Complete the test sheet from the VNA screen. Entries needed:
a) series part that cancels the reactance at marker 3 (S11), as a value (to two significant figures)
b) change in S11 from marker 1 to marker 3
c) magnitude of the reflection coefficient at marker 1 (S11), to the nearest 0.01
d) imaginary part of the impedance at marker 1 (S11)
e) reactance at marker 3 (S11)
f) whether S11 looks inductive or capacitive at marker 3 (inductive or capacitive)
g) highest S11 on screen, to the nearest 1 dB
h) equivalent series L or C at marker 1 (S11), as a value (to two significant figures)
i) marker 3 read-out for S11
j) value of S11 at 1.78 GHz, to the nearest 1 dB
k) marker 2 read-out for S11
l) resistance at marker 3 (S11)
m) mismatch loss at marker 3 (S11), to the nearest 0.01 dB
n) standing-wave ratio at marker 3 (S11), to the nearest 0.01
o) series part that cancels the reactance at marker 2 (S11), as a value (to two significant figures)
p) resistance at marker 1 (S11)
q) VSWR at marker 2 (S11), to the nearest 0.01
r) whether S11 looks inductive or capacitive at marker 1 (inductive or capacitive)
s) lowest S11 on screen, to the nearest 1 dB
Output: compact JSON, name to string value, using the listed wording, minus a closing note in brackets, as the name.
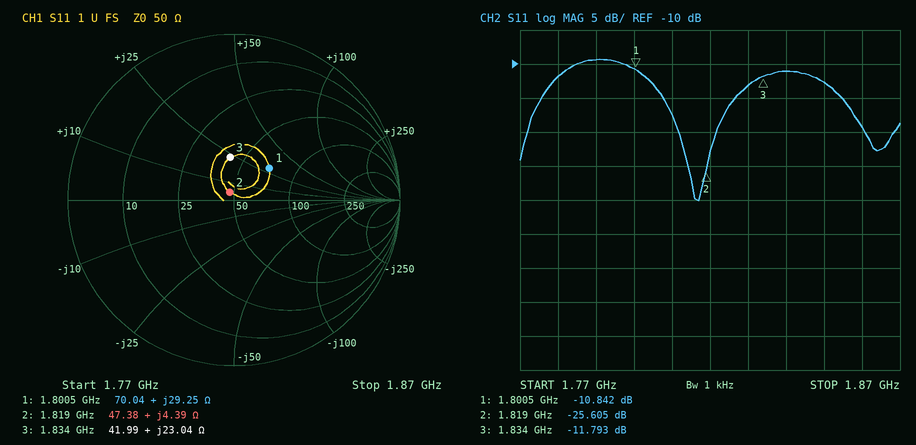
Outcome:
{"series part that cancels the reactance at marker 3 (S11), as a value": "3.8 pF", "change in S11 from marker 1 to marker 3": "-0.951 dB", "magnitude of the reflection coefficient at marker 1 (S11), to the nearest 0.01": "0.29", "imaginary part of the impedance at marker 1": "+29.25 Ω", "reactance at marker 3": "+23.04 Ω", "whether S11 looks inductive or capacitive at marker 3": "inductive", "highest S11 on screen, to the nearest 1 dB": "-9 dB", "equivalent series L or C at marker 1 (S11), as a value": "2.6 nH", "marker 3 read-out for S11": "-11.793 dB", "value of S11 at 1.78 GHz, to the nearest 1 dB": "-12 dB", "marker 2 read-out for S11": "-25.605 dB", "resistance at marker 3": "41.99 Ω", "mismatch loss at marker 3 (S11), to the nearest 0.01 dB": "0.30 dB", "standing-wave ratio at marker 3 (S11), to the nearest 0.01": "1.69", "series part that cancels the reactance at marker 2 (S11), as a value": "20 pF", "resistance at marker 1": "70.04 Ω", "VSWR at marker 2 (S11), to the nearest 0.01": "1.11", "whether S11 looks inductive or capacitive at marker 1": "inductive", "lowest S11 on screen, to the nearest 1 dB": "-30 dB"}
